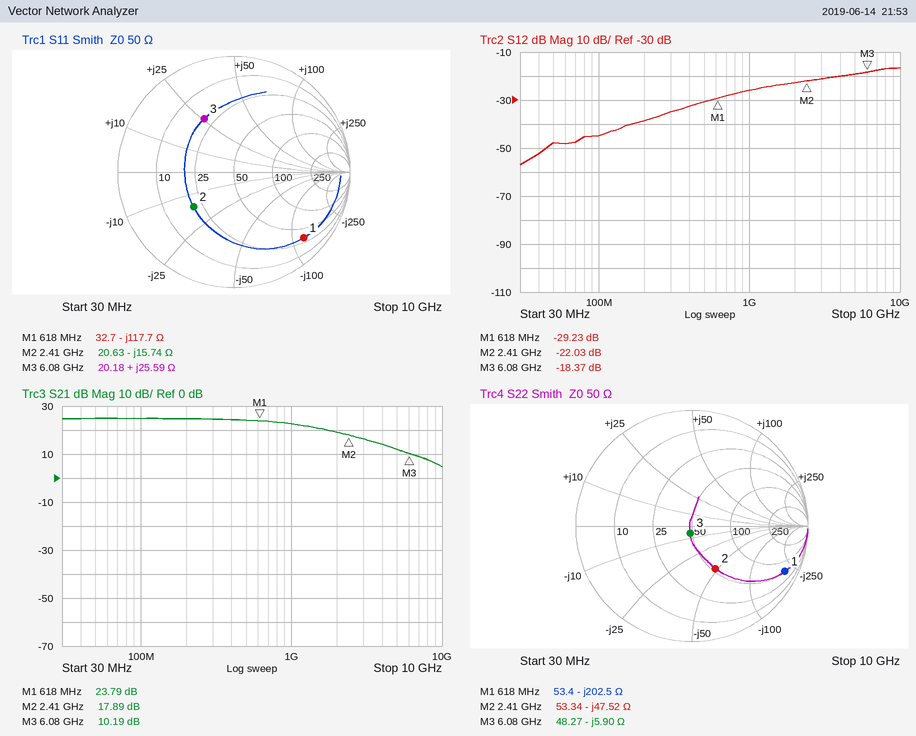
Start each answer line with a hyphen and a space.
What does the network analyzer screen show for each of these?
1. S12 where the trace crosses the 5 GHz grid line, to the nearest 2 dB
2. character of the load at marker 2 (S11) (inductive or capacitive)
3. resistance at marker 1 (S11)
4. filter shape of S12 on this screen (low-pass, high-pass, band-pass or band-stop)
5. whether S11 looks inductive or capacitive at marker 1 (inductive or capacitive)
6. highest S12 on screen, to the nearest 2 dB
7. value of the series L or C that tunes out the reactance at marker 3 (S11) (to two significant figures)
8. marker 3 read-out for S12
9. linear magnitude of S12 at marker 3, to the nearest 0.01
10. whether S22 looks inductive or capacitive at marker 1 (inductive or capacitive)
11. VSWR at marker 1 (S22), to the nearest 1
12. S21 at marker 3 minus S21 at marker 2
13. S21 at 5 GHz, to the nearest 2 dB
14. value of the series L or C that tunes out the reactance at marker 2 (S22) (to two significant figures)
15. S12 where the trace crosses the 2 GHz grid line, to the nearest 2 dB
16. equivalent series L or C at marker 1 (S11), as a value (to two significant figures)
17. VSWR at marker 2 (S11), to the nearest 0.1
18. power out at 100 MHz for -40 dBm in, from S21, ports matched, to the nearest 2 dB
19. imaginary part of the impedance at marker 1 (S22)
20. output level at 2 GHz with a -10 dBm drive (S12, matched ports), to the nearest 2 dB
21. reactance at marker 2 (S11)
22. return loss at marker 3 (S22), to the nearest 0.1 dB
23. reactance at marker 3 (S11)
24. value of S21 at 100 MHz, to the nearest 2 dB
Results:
- -20 dB
- capacitive
- 32.7 Ω
- high-pass
- capacitive
- -16 dB
- 1.0 pF
- -18.37 dB
- 0.12
- capacitive
- 17
- -7.70 dB
- 12 dB
- 3.1 nH
- -22 dB
- 2.2 pF
- 2.7
- -16 dBm
- -202.5 Ω
- -32 dBm
- -15.74 Ω
- 24.1 dB
- +25.59 Ω
- 24 dB
